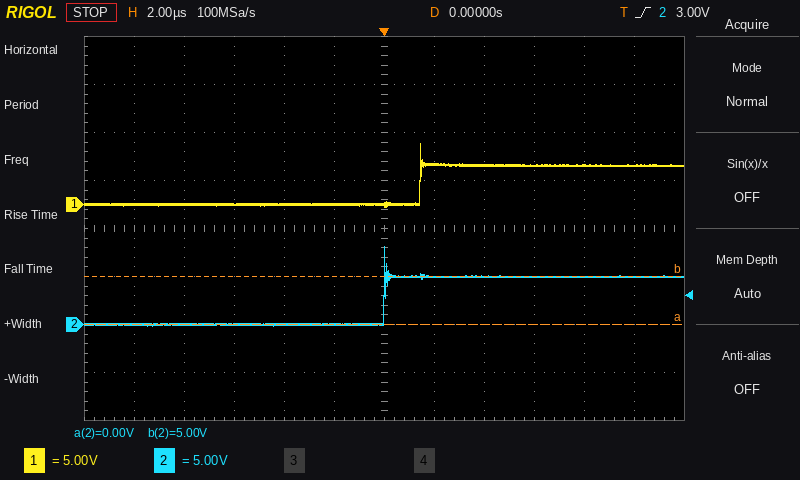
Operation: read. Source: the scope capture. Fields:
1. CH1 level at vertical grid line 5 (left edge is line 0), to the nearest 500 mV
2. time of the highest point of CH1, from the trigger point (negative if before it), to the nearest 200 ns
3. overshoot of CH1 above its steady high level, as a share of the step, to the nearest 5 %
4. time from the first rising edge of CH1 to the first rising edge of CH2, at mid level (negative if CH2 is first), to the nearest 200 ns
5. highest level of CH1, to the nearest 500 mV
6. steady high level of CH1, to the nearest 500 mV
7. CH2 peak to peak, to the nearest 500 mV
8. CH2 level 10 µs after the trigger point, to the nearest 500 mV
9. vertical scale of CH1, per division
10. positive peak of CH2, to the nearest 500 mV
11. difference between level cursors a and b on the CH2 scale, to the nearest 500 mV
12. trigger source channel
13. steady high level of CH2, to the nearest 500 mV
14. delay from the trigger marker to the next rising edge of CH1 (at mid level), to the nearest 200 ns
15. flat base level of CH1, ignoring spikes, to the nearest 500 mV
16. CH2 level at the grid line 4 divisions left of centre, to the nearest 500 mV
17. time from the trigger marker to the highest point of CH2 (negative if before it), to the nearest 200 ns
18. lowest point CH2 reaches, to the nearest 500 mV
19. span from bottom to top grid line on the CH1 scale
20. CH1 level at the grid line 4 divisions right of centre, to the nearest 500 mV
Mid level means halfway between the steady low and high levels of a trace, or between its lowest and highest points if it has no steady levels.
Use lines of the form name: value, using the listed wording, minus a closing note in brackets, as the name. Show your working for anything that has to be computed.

CH1 level at vertical grid line 5 (left edge is line 0), to the nearest 500 mV: 0.0 V
time of the highest point of CH1, from the trigger point (negative if before it), to the nearest 200 ns: +1.4 µs
overshoot of CH1 above its steady high level, as a share of the step, to the nearest 5 %: 55 %
time from the first rising edge of CH1 to the first rising edge of CH2, at mid level (negative if CH2 is first), to the nearest 200 ns: -1.4 µs
highest level of CH1, to the nearest 500 mV: 6.5 V
steady high level of CH1, to the nearest 500 mV: 4.0 V
CH2 peak to peak, to the nearest 500 mV: 8.0 V − (0.0 V) = 8.0 V
CH2 level 10 µs after the trigger point, to the nearest 500 mV: 5.0 V
vertical scale of CH1, per division: 5 V
positive peak of CH2, to the nearest 500 mV: 8.0 V
difference between level cursors a and b on the CH2 scale, to the nearest 500 mV: 5.0 V
trigger source channel: CH2
steady high level of CH2, to the nearest 500 mV: 5.0 V
delay from the trigger marker to the next rising edge of CH1 (at mid level), to the nearest 200 ns: 1.4 µs
flat base level of CH1, ignoring spikes, to the nearest 500 mV: 0.0 V
CH2 level at the grid line 4 divisions left of centre, to the nearest 500 mV: 0.0 V
time from the trigger marker to the highest point of CH2 (negative if before it), to the nearest 200 ns: 0.0 µs
lowest point CH2 reaches, to the nearest 500 mV: 0.0 V
span from bottom to top grid line on the CH1 scale: 40 V
CH1 level at the grid line 4 divisions right of centre, to the nearest 500 mV: 4.0 V
